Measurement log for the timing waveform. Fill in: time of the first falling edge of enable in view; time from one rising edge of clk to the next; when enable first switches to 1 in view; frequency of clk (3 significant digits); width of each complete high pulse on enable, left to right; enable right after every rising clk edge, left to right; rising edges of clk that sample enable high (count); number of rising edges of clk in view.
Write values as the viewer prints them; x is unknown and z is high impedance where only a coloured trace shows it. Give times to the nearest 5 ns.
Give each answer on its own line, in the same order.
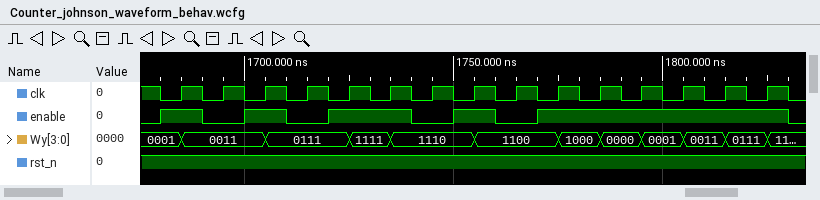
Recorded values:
1690 ns
10 ns
1680 ns
100 MHz
10 ns, 10 ns, 20 ns, 10 ns, 60 ns
1 0 1 0 1 1 0 1 0 1 1 1 1 1 1
11
15
